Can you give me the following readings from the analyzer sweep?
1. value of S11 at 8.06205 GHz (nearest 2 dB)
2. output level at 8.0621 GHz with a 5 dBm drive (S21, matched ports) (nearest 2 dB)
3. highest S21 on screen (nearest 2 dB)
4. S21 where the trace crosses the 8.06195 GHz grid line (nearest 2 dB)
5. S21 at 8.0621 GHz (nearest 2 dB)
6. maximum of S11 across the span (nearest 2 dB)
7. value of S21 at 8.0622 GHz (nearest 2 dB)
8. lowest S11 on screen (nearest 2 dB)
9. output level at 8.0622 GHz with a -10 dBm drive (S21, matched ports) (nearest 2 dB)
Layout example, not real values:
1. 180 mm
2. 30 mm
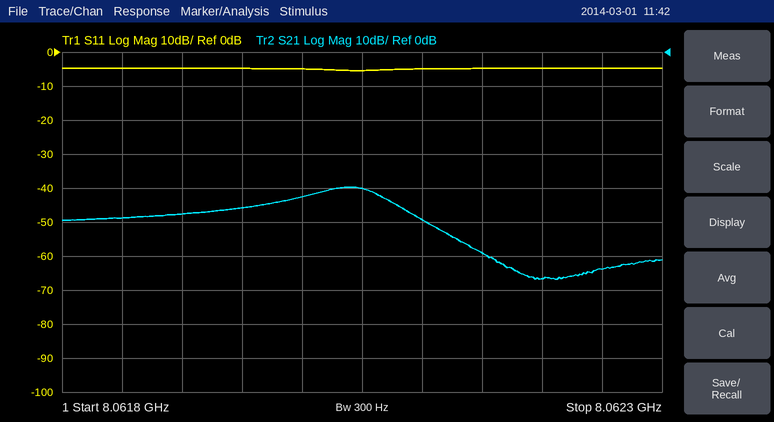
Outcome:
1. -6 dB
2. -44 dBm
3. -40 dB
4. -46 dB
5. -50 dB
6. -4 dB
7. -66 dB
8. -6 dB
9. -76 dBm
